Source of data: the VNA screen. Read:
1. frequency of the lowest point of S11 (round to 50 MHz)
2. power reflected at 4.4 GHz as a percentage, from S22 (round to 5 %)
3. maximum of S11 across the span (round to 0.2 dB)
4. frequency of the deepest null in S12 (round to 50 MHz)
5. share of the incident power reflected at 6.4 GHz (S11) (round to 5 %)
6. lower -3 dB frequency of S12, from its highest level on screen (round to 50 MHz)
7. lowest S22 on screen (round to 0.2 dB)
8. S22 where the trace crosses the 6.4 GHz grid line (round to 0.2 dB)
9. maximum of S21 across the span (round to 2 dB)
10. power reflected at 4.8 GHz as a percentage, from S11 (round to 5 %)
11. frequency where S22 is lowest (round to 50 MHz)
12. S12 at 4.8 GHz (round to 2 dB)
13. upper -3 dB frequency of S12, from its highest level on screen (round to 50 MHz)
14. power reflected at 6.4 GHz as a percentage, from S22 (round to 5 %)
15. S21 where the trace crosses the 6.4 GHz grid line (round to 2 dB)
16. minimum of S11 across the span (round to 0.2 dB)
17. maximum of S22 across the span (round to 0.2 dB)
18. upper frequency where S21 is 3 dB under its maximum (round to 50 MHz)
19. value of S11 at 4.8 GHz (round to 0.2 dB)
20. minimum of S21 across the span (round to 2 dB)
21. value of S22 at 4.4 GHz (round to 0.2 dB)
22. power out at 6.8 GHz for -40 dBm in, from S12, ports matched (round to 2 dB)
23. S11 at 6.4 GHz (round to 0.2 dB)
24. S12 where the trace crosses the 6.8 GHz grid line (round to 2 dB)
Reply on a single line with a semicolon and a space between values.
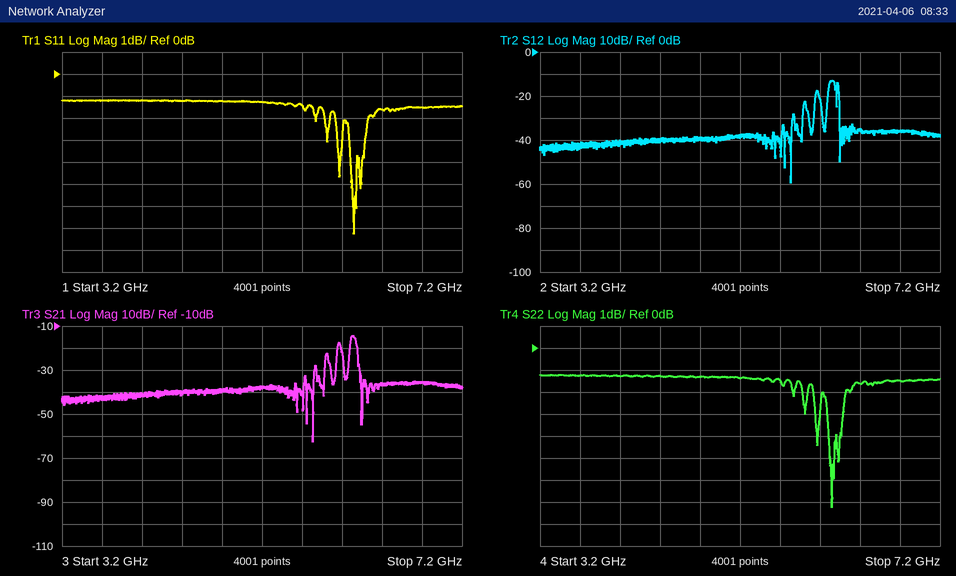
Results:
6.10 GHz; 75 %; -1.2 dB; 5.70 GHz; 70 %; 6.10 GHz; -7.2 dB; -1.6 dB; -14 dB; 75 %; 6.10 GHz; -40 dB; 6.15 GHz; 70 %; -36 dB; -7.2 dB; -1.2 dB; 6.15 GHz; -1.2 dB; -62 dB; -1.2 dB; -76 dBm; -1.6 dB; -36 dB
